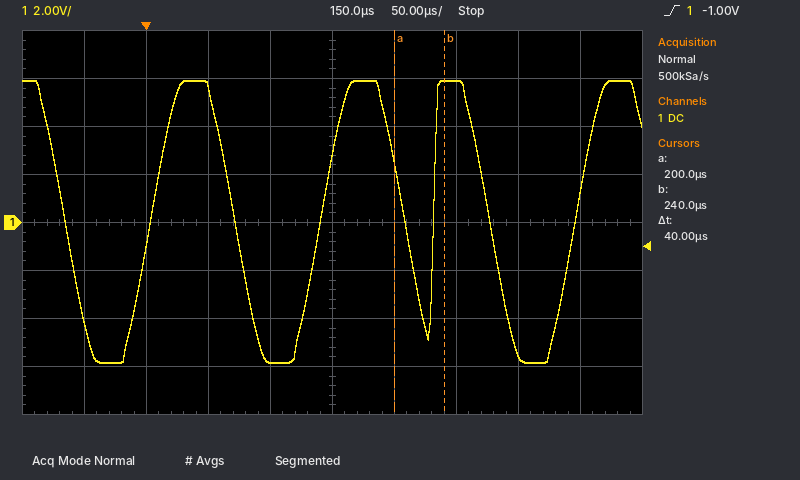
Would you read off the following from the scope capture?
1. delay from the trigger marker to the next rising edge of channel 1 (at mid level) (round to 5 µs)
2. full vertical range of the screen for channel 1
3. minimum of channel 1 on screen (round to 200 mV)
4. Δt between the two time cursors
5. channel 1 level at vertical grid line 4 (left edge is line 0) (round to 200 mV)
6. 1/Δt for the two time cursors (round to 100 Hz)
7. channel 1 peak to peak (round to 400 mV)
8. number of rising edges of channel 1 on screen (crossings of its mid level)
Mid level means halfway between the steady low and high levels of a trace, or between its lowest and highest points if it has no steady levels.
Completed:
5 µs
16 V
-5.8 V
40 µs
-5.8 V
25.0 kHz
11.6 V
4
